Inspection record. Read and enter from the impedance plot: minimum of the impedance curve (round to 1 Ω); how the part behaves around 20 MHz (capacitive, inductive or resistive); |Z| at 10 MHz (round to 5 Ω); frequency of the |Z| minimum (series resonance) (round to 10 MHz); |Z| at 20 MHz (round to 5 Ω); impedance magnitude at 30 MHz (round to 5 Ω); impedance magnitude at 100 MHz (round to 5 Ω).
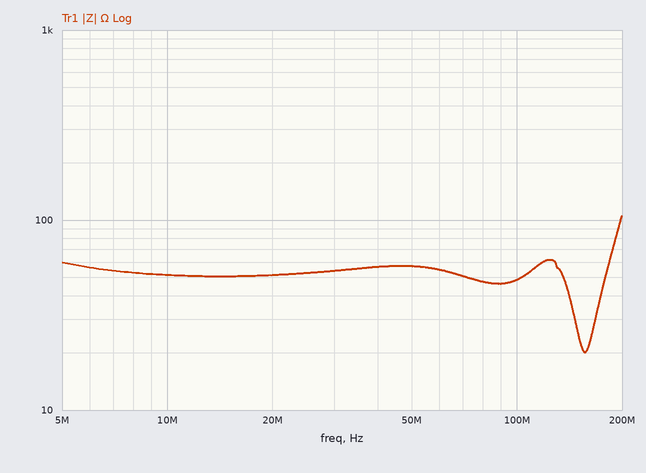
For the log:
20 Ω
resistive
50 Ω
160 MHz
50 Ω
55 Ω
50 Ω
